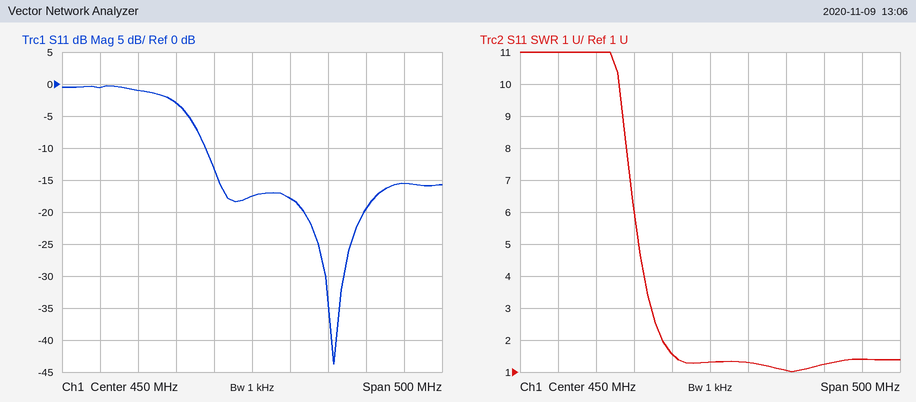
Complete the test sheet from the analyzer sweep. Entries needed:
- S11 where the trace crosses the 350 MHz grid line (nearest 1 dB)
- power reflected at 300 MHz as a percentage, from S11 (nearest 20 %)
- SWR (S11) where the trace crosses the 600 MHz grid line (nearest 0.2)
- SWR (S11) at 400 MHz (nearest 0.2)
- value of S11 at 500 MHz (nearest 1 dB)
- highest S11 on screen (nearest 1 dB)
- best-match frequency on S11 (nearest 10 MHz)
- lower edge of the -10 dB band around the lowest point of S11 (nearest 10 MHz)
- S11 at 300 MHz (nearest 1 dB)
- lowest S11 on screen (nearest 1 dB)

-3 dB
80 %
1.2
1.6
-18 dB
0 dB
560 MHz
390 MHz
-1 dB
-44 dB
